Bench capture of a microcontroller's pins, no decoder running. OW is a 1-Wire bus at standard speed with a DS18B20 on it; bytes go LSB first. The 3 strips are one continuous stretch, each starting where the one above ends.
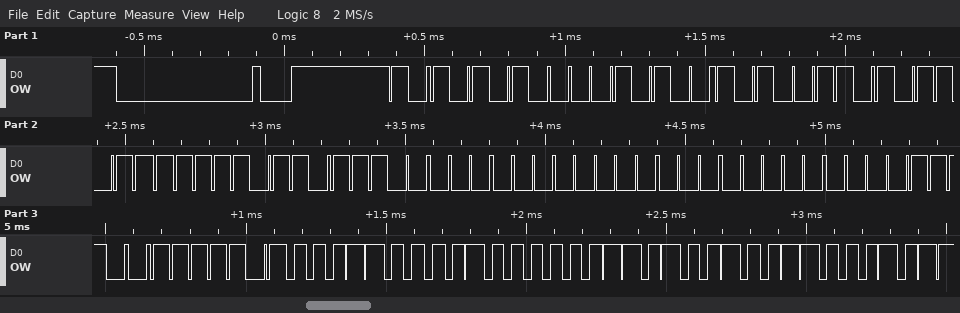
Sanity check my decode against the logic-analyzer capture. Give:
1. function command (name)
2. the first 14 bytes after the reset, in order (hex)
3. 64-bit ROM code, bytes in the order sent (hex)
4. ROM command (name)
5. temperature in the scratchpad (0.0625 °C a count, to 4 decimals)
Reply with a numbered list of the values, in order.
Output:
1. Read Scratchpad
2. 55 28 65 ED 6F 07 00 00 70 BE 18 02 4B 46
3. 28 65 ED 6F 07 00 00 70
4. Match ROM
5. 33.5000 °C
